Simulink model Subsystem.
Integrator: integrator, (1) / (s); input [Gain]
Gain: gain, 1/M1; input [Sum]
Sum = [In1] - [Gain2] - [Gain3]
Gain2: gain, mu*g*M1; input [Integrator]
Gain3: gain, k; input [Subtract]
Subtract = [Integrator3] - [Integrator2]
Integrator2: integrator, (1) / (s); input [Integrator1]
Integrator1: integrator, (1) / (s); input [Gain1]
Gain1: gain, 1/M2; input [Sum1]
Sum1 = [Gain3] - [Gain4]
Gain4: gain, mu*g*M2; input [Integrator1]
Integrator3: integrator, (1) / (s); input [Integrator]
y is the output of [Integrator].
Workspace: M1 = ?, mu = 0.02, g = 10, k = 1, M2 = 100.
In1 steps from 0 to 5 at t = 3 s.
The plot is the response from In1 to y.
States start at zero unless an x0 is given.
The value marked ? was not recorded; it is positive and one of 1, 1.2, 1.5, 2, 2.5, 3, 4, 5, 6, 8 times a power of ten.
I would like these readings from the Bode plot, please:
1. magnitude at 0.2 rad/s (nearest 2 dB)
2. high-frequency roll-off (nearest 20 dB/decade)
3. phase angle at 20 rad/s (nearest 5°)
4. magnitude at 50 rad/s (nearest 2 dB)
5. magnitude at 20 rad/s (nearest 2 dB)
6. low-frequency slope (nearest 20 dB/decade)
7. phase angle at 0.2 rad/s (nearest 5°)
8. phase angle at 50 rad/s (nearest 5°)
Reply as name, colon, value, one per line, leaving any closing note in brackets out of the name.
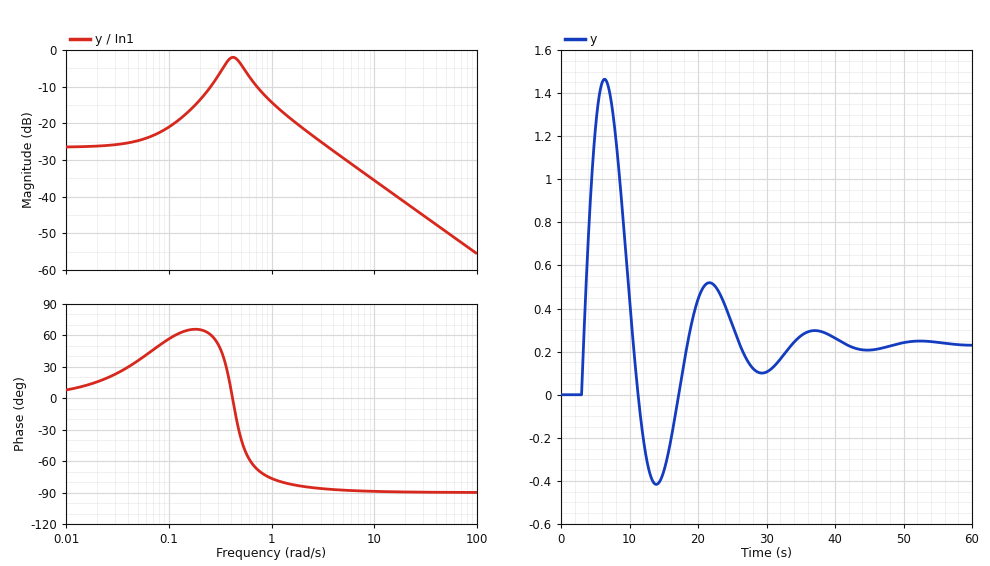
magnitude at 0.2 rad/s: -14 dB
high-frequency roll-off: -20 dB/decade
phase angle at 20 rad/s: -90°
magnitude at 50 rad/s: -50 dB
magnitude at 20 rad/s: -42 dB
low-frequency slope: 0 dB/decade
phase angle at 0.2 rad/s: 65°
phase angle at 50 rad/s: -90°
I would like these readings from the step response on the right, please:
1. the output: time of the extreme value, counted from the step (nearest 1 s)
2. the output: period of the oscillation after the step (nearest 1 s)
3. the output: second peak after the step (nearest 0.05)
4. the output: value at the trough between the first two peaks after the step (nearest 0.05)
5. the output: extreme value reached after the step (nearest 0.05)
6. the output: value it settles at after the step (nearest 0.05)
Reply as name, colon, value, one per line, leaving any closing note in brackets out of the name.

the output: time of the extreme value, counted from the step: 3 s
the output: period of the oscillation after the step: 15 s
the output: second peak after the step: 0.50
the output: value at the trough between the first two peaks after the step: -0.40
the output: extreme value reached after the step: 1.45
the output: value it settles at after the step: 0.25
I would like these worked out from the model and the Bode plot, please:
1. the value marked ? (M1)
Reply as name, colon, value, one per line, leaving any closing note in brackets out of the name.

the value marked ?: 6
